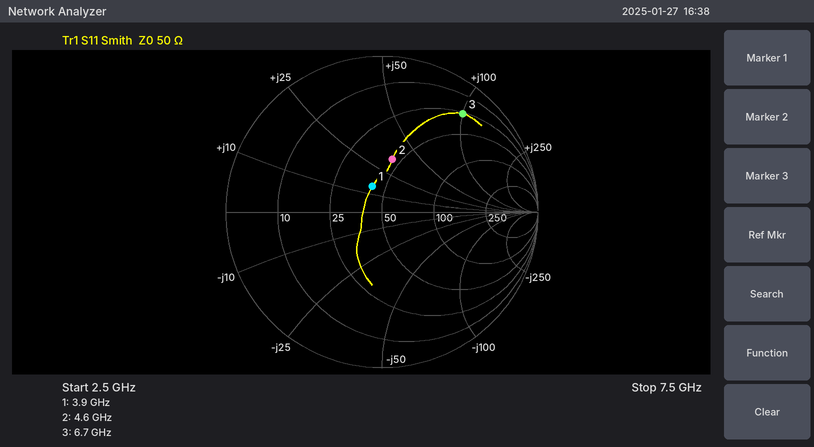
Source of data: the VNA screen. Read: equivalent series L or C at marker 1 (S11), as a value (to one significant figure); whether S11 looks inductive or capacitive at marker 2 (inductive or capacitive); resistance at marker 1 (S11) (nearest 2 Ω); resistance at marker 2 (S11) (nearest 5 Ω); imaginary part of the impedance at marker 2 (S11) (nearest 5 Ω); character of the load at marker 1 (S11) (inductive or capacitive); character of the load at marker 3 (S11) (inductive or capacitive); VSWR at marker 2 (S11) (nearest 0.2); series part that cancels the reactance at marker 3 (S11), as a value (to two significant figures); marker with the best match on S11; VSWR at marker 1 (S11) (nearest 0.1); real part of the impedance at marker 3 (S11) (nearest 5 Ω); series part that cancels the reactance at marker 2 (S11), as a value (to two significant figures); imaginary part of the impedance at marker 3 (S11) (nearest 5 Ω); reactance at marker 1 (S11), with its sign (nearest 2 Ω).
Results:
600 pH
inductive
42 Ω
45 Ω
+35 Ω
inductive
inductive
2.0
240 fF
marker 1
1.4
25 Ω
1.0 pF
+100 Ω
+14 Ω
